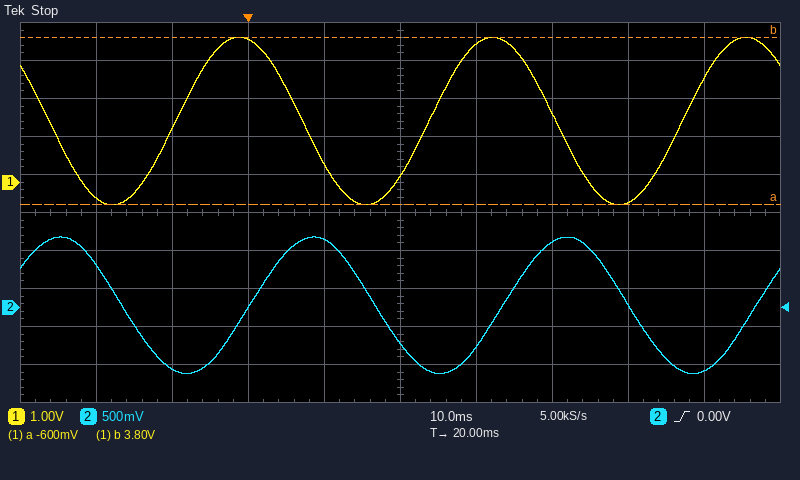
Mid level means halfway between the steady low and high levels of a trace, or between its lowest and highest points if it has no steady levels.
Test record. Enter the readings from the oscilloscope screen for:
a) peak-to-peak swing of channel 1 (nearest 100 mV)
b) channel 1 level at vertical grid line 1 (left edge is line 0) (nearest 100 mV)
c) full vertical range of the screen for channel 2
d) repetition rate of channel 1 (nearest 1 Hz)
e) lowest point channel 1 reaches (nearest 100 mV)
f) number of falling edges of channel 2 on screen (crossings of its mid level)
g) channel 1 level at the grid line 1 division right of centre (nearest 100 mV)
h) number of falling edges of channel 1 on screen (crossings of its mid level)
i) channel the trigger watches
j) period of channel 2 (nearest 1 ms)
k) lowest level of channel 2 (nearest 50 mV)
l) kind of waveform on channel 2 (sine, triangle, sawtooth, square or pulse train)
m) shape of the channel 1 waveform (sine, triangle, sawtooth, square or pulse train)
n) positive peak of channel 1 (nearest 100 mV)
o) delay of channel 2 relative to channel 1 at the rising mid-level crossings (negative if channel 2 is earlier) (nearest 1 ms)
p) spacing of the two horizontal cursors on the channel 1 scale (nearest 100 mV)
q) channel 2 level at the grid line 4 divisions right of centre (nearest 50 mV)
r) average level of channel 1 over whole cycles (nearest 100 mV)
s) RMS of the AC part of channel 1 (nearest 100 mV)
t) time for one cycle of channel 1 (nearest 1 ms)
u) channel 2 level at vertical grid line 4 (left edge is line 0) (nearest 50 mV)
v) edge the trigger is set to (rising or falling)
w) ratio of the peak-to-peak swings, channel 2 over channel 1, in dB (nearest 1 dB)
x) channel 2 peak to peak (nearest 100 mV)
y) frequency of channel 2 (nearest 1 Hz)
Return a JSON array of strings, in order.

["4.4 V", "-400 mV", "5 V", "30 Hz", "-600 mV", "3", "3.6 V", "3", "channel 2", "33 ms", "-850 mV", "sine", "sine", "3.8 V", "+10 ms", "4.4 V", "-850 mV", "1.6 V", "1.6 V", "33 ms", "900 mV", "rising", "-8 dB", "1.80 V", "30 Hz"]
